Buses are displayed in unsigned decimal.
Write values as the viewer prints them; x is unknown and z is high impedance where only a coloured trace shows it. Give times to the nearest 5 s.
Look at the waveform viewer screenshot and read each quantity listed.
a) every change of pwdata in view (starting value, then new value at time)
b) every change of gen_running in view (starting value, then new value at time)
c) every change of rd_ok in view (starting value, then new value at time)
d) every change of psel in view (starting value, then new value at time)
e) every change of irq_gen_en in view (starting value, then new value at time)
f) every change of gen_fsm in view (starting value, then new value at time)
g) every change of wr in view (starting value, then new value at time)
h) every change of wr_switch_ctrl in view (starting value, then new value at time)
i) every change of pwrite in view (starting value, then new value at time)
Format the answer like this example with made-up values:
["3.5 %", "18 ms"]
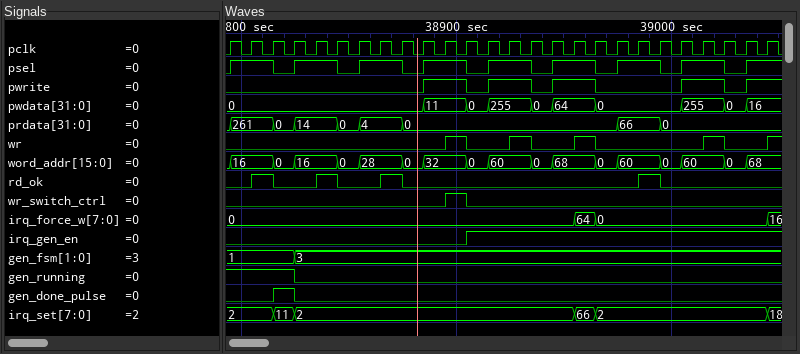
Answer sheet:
["0, 11 at 38885 s, 0 at 38905 s, 255 at 38915 s, 0 at 38935 s, 64 at 38945 s, 0 at 38965 s, 255 at 39005 s, 0 at 39025 s, 16 at 39035 s", "1, 0 at 38825 s", "0, 1 at 38805 s, 0 at 38815 s, 1 at 38835 s, 0 at 38845 s, 1 at 38865 s, 0 at 38875 s, 1 at 38985 s, 0 at 38995 s", "0, 1 at 38795 s, 0 at 38815 s, 1 at 38825 s, 0 at 38845 s, 1 at 38855 s, 0 at 38875 s, 1 at 38885 s, 0 at 38905 s, 1 at 38915 s, 0 at 38935 s, 1 at 38945 s, 0 at 38965 s, 1 at 38975 s, 0 at 38995 s, 1 at 39005 s, 0 at 39025 s, 1 at 39035 s", "0, 1 at 38905 s", "1, 3 at 38825 s", "0, 1 at 38895 s, 0 at 38905 s, 1 at 38925 s, 0 at 38935 s, 1 at 38955 s, 0 at 38965 s, 1 at 39015 s, 0 at 39025 s, 1 at 39045 s", "0, 1 at 38895 s, 0 at 38905 s", "0, 1 at 38885 s, 0 at 38905 s, 1 at 38915 s, 0 at 38935 s, 1 at 38945 s, 0 at 38965 s, 1 at 39005 s, 0 at 39025 s, 1 at 39035 s"]
